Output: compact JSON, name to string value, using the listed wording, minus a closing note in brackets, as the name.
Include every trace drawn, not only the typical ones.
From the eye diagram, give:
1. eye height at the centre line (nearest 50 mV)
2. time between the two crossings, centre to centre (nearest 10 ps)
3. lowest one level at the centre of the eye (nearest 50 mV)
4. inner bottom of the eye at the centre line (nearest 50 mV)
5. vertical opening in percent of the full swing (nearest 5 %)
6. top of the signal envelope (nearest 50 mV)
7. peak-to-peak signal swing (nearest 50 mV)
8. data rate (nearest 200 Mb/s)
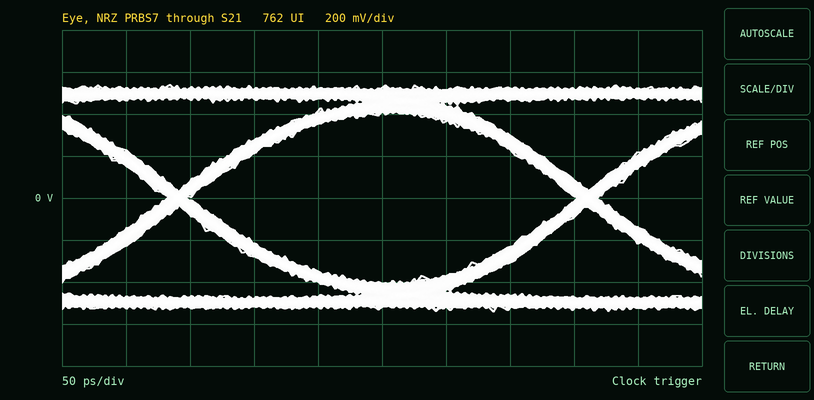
{"eye height at the centre line": "800 mV", "time between the two crossings, centre to centre": "320 ps", "lowest one level at the centre of the eye": "400 mV", "inner bottom of the eye at the centre line": "-400 mV", "vertical opening in percent of the full swing": "75 %", "top of the signal envelope": "550 mV", "peak-to-peak signal swing": "1.10 V", "data rate": "3.2 Gb/s"}
